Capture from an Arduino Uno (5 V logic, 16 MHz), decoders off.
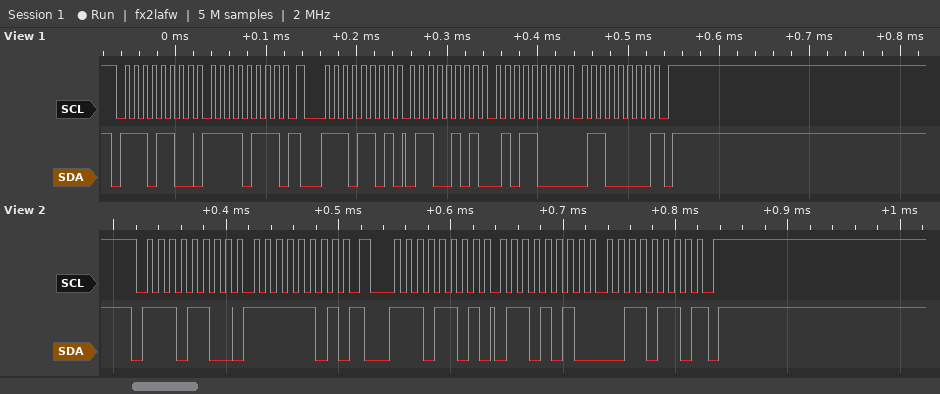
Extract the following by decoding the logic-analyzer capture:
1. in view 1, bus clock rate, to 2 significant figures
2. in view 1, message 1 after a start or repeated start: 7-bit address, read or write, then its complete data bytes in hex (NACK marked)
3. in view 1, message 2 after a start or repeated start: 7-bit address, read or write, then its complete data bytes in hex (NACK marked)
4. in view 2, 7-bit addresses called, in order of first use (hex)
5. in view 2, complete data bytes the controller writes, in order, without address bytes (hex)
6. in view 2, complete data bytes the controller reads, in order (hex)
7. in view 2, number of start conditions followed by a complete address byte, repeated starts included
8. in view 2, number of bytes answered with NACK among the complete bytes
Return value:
100 kHz
0x76 write: F7
0x76 read: 65 58 60 NACK
0x76
FD
6A 36
2
1
